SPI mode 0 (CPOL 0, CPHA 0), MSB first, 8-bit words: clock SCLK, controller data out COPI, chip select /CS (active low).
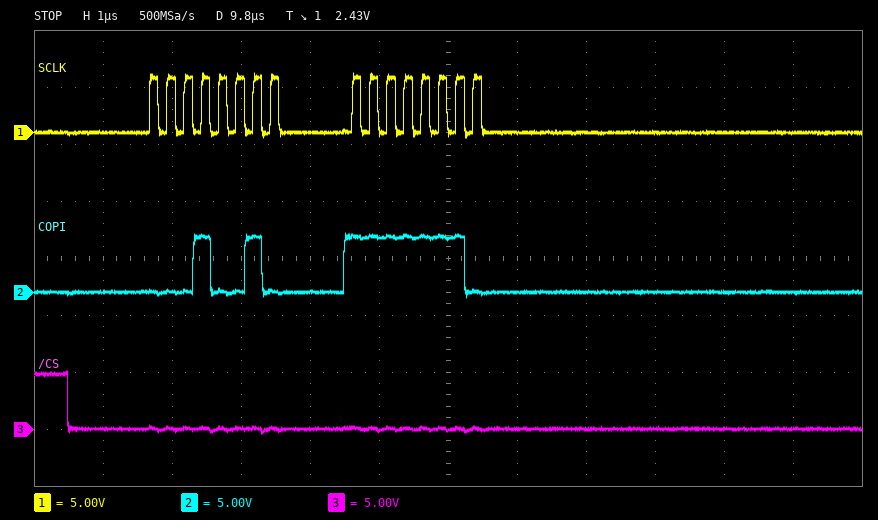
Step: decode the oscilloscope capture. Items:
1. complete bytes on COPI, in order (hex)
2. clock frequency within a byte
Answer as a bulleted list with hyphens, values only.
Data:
- 12 FE
- 4 MHz
